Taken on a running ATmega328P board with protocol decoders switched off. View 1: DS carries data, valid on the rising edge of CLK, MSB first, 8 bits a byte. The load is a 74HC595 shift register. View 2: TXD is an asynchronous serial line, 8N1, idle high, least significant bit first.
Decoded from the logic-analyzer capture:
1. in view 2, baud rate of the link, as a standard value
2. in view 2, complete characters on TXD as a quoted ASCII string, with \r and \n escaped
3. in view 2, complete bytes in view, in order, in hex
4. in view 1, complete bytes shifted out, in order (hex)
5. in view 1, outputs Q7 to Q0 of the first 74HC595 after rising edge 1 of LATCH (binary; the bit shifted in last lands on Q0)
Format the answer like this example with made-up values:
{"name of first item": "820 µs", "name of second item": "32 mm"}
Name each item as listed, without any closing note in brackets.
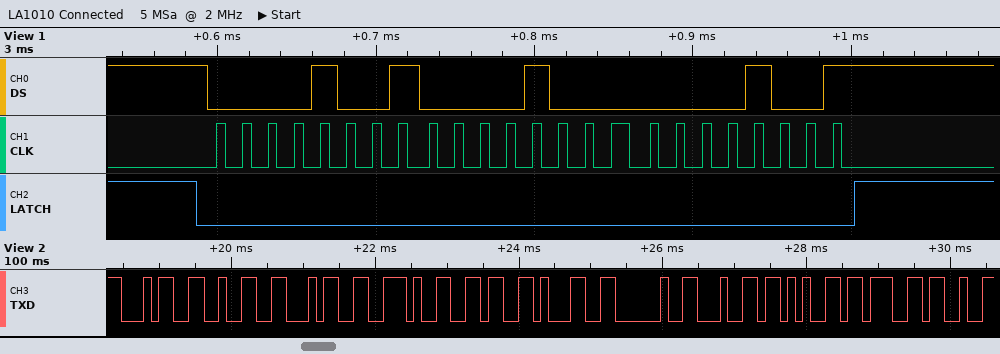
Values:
{"in view 2, baud rate of the link, as a standard value": "9600 baud", "in view 2, complete characters on TXD as a quoted ASCII string, with \\r and \\n escaped": "\"424.61 deg\"", "in view 2, complete bytes in view, in order, in hex": "0x34 0x32 0x34 0x2E 0x36 0x31 0x20 0x64 0x65 0x67", "in view 1, complete bytes shifted out, in order": "09 08 09", "in view 1, outputs Q7 to Q0 of the first 74HC595 after rising edge 1 of LATCH": "00001001"}
